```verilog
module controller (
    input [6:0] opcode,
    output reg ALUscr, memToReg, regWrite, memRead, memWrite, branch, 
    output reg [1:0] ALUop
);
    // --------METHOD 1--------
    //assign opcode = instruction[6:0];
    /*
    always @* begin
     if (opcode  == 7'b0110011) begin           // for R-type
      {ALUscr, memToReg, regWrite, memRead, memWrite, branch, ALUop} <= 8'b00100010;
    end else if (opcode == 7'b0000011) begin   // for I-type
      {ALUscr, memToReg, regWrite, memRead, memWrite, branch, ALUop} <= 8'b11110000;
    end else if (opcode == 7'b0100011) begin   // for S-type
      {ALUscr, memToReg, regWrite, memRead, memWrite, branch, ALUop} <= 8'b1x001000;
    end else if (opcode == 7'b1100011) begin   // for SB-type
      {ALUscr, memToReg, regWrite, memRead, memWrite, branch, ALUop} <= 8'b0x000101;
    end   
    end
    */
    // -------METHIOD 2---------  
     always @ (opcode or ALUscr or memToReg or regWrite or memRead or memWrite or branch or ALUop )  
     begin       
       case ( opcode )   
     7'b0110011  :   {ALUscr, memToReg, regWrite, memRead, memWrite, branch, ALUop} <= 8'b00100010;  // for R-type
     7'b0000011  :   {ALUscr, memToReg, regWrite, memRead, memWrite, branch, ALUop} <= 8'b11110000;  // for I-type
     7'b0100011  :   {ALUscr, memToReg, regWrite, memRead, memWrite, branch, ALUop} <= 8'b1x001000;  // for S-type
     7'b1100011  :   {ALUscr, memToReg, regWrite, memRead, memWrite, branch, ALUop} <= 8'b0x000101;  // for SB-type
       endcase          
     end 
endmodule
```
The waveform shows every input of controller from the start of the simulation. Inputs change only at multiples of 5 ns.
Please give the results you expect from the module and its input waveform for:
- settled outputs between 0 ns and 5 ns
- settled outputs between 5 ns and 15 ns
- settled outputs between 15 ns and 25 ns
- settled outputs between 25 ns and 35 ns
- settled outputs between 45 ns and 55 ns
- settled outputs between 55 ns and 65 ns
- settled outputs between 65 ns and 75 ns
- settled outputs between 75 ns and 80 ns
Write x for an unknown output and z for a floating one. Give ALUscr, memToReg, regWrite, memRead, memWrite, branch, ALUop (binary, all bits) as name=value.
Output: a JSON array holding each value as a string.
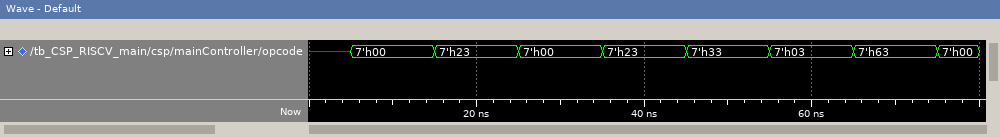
["ALUscr=x, memToReg=x, regWrite=x, memRead=x, memWrite=x, branch=x, ALUop=x", "ALUscr=x, memToReg=x, regWrite=x, memRead=x, memWrite=x, branch=x, ALUop=x", "ALUscr=1, memToReg=x, regWrite=0, memRead=0, memWrite=1, branch=0, ALUop=00", "ALUscr=1, memToReg=x, regWrite=0, memRead=0, memWrite=1, branch=0, ALUop=00", "ALUscr=0, memToReg=0, regWrite=1, memRead=0, memWrite=0, branch=0, ALUop=10", "ALUscr=1, memToReg=1, regWrite=1, memRead=1, memWrite=0, branch=0, ALUop=00", "ALUscr=0, memToReg=x, regWrite=0, memRead=0, memWrite=0, branch=1, ALUop=01", "ALUscr=0, memToReg=x, regWrite=0, memRead=0, memWrite=0, branch=1, ALUop=01"]
